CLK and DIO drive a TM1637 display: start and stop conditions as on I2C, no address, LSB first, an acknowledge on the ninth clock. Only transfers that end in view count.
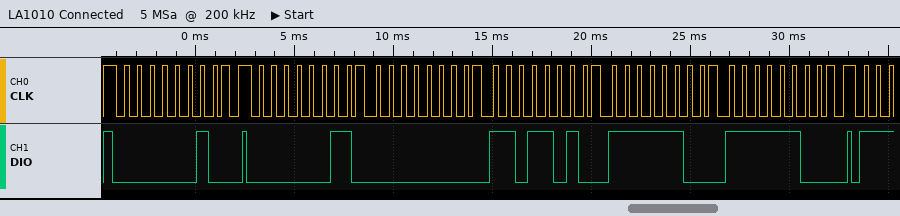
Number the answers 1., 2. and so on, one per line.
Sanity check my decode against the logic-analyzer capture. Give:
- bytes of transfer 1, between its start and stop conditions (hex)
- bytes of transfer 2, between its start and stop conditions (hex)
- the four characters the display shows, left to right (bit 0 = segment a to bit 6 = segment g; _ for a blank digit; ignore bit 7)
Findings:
1. 40
2. C0 00 5B 3F 3F
3. _200
